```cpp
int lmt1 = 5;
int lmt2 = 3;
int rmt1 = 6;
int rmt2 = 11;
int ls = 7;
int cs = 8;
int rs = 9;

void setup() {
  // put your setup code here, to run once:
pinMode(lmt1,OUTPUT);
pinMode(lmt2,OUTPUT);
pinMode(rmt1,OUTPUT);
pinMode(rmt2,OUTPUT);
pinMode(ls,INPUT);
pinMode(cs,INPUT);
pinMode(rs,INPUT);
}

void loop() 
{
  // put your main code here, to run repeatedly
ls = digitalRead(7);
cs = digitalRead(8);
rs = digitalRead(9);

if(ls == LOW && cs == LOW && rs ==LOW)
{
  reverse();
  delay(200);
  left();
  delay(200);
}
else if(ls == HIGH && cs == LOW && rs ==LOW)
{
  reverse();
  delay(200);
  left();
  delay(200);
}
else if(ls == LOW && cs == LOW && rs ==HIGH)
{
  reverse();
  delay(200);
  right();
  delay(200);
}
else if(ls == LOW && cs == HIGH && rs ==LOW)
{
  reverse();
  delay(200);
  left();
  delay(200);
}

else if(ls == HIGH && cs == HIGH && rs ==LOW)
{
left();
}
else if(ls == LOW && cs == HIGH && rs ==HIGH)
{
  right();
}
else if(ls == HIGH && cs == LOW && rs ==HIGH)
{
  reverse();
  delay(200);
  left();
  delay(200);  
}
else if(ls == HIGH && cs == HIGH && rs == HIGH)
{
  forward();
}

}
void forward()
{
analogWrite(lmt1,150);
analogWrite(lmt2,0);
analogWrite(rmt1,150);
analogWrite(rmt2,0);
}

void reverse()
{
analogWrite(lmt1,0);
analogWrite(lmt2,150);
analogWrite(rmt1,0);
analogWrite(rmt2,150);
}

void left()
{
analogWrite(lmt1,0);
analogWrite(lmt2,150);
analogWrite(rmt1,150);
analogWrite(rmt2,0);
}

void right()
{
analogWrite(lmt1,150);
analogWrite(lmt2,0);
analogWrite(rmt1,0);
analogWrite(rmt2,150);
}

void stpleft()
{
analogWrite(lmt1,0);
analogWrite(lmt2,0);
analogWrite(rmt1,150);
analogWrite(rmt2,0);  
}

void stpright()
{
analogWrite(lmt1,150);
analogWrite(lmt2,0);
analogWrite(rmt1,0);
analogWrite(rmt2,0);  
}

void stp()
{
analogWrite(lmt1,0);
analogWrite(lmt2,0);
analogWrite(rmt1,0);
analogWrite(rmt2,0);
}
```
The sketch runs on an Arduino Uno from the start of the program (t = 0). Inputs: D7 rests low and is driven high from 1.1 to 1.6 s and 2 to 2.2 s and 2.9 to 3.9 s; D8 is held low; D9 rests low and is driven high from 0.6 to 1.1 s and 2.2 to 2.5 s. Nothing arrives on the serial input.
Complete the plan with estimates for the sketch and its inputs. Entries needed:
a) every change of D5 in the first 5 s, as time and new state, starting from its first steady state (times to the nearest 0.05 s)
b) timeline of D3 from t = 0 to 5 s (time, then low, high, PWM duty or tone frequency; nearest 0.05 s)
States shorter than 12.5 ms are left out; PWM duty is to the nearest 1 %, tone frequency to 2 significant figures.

0 s low; 1 s PWM 59 %; 1.2 s low; 2.6 s PWM 59 %; 2.8 s low
0 s PWM 59 %; 1 s low; 1.2 s PWM 59 %; 2.6 s low; 2.8 s PWM 59 %
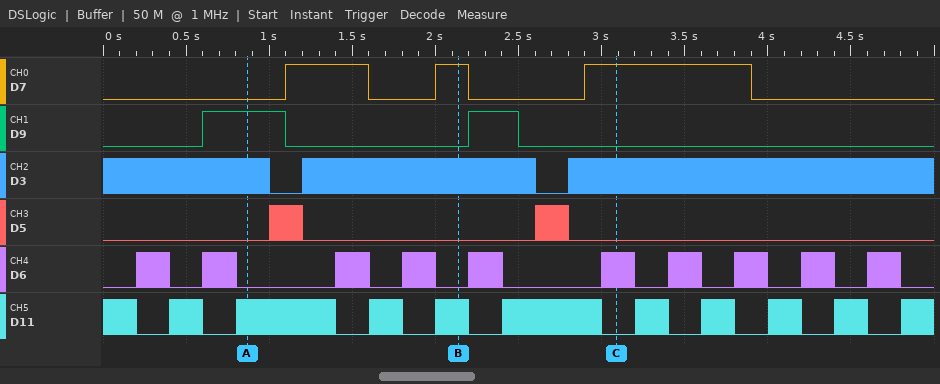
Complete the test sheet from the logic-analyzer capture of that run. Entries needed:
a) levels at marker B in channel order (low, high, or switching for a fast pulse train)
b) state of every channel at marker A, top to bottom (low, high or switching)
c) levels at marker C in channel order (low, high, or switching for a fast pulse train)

D7 high, D9 low, D3 switching, D5 low, D6 low, D11 switching
D7 low, D9 high, D3 switching, D5 low, D6 low, D11 switching
D7 high, D9 low, D3 switching, D5 low, D6 switching, D11 low
